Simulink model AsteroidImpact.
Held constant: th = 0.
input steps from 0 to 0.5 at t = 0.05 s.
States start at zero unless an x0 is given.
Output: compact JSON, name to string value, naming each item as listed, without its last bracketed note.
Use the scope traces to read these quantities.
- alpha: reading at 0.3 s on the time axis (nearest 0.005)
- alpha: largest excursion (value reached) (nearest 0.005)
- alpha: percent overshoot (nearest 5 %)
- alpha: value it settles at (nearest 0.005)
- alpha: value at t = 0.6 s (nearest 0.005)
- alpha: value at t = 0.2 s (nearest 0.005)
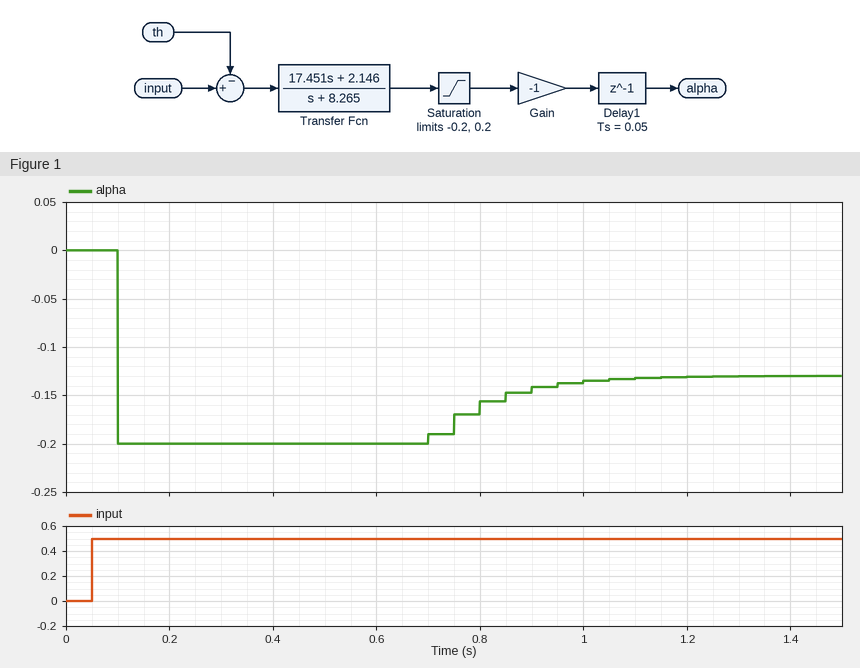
{"alpha: reading at 0.3 s on the time axis": "-0.200", "alpha: largest excursion (value reached)": "-0.200", "alpha: percent overshoot": "55 %", "alpha: value it settles at": "-0.130", "alpha: value at t = 0.6 s": "-0.200", "alpha: value at t = 0.2 s": "-0.200"}
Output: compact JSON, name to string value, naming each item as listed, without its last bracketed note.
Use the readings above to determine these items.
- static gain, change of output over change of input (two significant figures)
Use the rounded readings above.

{"static gain, change of output over change of input": "-0.26"}
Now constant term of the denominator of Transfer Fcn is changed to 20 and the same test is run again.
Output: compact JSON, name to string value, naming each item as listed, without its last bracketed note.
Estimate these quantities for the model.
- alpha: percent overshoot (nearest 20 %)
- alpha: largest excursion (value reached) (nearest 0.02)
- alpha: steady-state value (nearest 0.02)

{"alpha: percent overshoot": "280 %", "alpha: largest excursion (value reached)": "-0.20", "alpha: steady-state value": "-0.06"}
